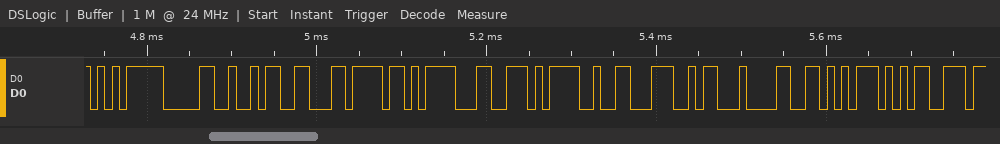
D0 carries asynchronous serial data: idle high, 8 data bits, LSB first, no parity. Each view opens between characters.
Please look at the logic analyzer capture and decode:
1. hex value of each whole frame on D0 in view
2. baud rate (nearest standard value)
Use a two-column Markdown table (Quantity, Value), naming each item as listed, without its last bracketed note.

| Quantity | Value |
|---|---|
| hex value of each whole frame on D0 in view | F5, 30, 9A, EC, EB, CC, 3D, C6, 1A, 98, 75, CD |
| baud rate | 115200 baud |
